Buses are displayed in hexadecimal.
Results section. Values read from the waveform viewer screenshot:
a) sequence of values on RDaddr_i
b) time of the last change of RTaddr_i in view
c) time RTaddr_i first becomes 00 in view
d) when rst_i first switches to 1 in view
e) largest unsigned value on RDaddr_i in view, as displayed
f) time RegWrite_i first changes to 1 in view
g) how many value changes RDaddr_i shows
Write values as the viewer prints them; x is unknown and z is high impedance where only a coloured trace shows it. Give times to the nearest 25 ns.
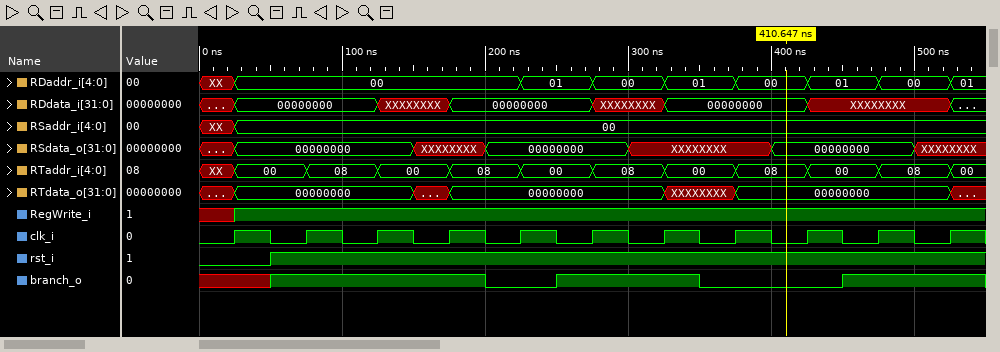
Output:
XX, 00, 01, 00, 01, 00, 01, 00, 01
525 ns
25 ns
50 ns
01
25 ns
8
